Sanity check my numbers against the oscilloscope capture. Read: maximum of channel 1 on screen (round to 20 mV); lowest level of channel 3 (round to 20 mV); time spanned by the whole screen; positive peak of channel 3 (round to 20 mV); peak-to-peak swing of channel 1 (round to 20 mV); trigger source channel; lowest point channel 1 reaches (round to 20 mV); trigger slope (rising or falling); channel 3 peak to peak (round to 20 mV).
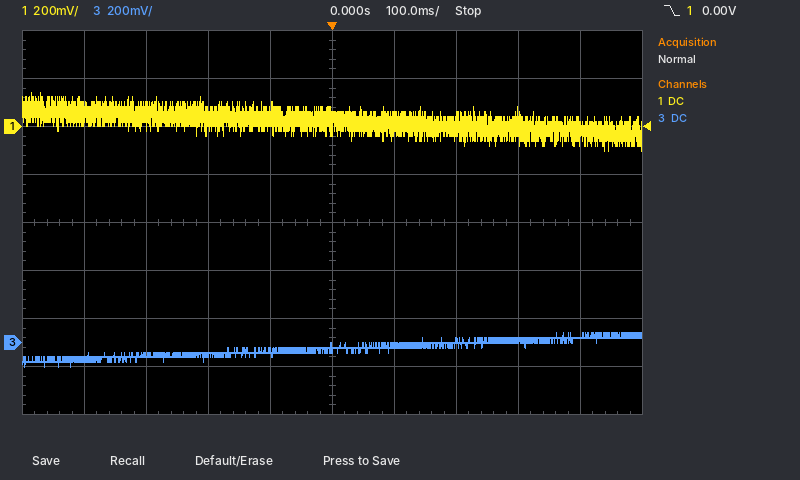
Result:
140 mV
-100 mV
1 s
40 mV
240 mV
channel 1
-100 mV
falling
140 mV
